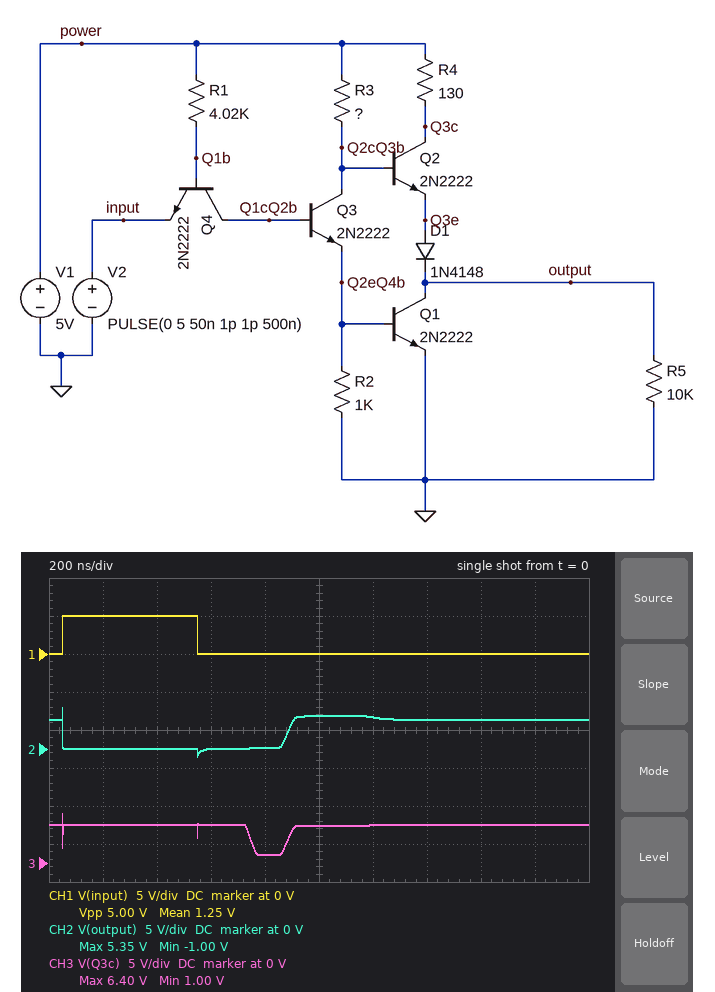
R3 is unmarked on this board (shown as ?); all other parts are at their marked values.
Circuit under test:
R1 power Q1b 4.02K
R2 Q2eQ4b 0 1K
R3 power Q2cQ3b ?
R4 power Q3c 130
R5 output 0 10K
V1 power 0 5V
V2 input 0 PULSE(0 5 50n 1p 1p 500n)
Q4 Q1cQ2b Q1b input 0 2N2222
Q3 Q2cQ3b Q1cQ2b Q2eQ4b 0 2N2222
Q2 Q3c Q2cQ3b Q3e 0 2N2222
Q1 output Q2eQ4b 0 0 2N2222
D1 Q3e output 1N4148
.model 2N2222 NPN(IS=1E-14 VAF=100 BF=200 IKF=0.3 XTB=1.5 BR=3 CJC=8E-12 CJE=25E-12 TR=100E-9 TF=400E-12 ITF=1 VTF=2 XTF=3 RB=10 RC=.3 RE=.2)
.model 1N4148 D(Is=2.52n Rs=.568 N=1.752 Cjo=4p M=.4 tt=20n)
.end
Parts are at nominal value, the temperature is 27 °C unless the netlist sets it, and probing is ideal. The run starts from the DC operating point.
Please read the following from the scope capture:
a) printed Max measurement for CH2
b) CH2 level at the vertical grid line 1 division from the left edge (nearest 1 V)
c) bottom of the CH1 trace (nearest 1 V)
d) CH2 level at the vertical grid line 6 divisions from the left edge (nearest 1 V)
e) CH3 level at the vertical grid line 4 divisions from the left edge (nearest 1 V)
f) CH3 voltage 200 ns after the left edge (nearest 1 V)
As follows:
5.35 V
0 V
0 V
4 V
1 V
5 V
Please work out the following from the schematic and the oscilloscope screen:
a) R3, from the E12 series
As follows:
3.3 kΩ
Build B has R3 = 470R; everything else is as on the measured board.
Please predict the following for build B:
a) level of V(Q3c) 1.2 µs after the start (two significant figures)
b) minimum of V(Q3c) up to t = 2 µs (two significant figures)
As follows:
970 mV
900 mV
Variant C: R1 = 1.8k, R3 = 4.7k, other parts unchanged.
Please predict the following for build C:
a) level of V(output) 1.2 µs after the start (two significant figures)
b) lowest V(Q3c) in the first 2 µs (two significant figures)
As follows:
3.8 V
1.4 V
